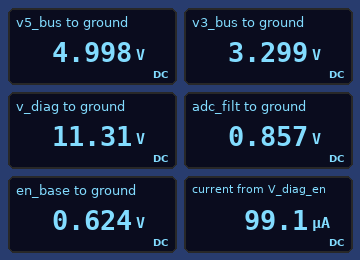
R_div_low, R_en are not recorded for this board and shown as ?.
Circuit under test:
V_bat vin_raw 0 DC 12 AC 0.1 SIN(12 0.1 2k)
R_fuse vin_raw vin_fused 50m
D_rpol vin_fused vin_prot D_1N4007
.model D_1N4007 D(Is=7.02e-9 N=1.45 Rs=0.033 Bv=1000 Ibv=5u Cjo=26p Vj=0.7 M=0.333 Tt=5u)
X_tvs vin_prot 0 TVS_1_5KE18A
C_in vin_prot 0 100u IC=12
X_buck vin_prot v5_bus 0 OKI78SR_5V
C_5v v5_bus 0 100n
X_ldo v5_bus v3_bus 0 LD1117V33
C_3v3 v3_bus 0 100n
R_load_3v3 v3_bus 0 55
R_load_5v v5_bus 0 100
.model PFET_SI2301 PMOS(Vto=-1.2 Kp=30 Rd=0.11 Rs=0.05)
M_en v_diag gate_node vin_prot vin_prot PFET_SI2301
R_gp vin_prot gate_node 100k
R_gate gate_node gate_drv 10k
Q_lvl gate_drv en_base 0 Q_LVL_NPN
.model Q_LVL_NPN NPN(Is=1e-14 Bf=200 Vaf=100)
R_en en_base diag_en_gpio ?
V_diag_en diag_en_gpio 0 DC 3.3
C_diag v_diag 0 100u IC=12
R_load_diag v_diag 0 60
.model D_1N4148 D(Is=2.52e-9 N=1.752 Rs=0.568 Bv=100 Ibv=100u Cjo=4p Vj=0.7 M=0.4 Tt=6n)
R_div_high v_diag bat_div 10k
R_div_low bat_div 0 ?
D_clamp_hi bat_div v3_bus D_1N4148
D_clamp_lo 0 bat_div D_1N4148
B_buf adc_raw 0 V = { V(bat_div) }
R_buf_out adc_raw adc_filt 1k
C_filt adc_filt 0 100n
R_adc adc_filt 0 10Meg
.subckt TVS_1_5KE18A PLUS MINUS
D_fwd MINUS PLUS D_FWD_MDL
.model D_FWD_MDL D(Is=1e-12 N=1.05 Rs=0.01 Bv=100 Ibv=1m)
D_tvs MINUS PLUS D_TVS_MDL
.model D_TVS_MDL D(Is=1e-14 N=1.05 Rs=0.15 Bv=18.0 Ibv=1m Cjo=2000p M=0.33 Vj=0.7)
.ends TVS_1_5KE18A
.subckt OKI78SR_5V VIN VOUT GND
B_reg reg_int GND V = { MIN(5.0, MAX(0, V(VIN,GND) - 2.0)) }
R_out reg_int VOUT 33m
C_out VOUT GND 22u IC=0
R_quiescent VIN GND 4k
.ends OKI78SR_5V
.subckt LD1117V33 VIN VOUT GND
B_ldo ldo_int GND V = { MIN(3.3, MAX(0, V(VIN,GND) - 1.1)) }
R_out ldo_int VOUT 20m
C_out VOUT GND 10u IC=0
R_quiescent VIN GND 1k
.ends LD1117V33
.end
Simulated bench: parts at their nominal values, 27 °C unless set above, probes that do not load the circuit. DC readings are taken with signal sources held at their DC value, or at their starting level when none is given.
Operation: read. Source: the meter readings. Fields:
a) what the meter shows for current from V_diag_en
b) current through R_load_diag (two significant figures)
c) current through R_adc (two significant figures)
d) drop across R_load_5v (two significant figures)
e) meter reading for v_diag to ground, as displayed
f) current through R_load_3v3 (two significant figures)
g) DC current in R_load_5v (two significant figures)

99.1 µA
190 mA
86 nA
5.0 V
11.31 V
60 mA
50 mA
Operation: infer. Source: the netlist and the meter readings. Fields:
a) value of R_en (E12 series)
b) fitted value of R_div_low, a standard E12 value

27 kΩ
820 Ω
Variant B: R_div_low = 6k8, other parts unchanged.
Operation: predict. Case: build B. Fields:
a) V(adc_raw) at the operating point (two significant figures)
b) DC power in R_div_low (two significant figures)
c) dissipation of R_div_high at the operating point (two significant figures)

3.8 V
2.1 mW
5.6 mW
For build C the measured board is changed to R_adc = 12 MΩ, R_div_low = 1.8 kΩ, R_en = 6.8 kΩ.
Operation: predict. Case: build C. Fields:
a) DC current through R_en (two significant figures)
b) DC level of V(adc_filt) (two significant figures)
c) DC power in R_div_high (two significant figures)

390 µA
1.7 V
9.2 mW
